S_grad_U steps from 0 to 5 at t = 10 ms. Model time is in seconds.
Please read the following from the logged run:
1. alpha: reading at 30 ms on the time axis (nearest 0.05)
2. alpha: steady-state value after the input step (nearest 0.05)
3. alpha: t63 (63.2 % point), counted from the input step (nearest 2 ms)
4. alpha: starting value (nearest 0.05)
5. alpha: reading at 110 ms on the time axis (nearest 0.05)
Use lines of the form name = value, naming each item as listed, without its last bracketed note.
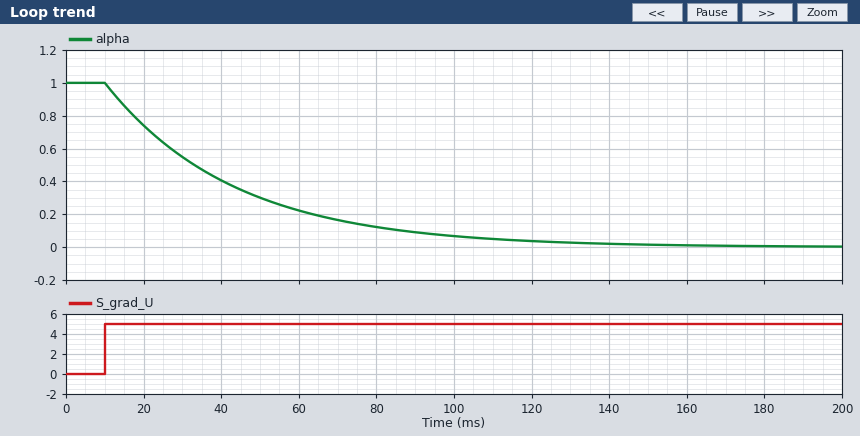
alpha: reading at 30 ms on the time axis = 0.55
alpha: steady-state value after the input step = 0.00
alpha: t63 (63.2 % point), counted from the input step = 34 ms
alpha: starting value = 1.00
alpha: reading at 110 ms on the time axis = 0.05
